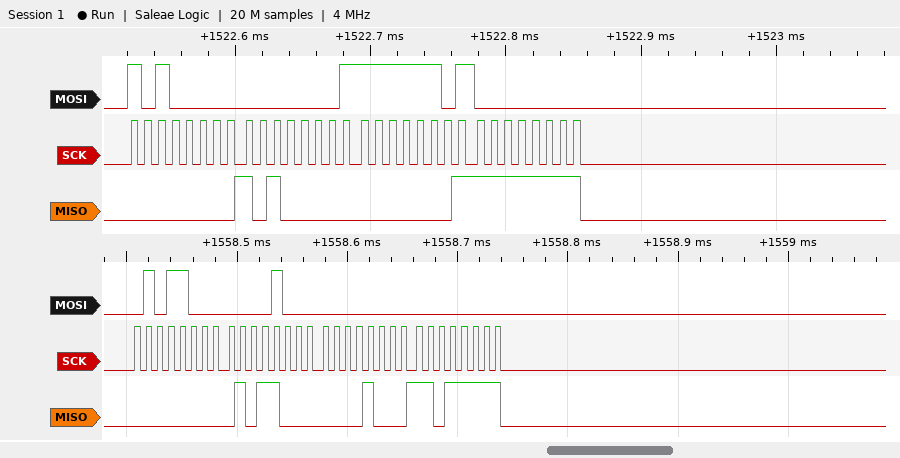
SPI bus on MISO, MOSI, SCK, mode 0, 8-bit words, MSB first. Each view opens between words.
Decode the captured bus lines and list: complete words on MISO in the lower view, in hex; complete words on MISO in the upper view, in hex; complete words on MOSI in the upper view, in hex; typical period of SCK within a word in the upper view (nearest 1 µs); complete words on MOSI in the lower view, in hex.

00, 58, 08, DF
00, A0, 01, FF
A0, 01, FD, 00
10 µs
58, 08, 00, 00
